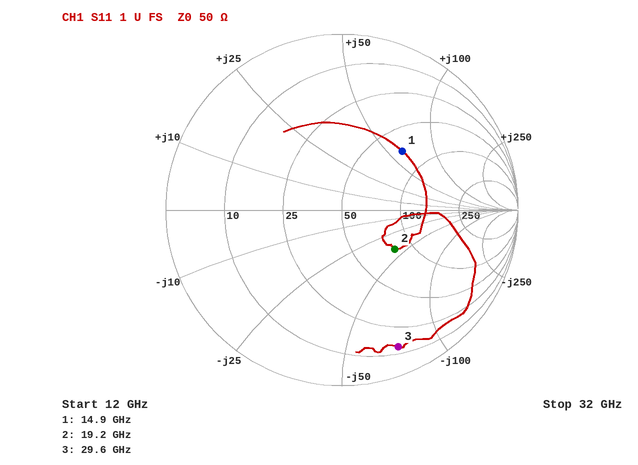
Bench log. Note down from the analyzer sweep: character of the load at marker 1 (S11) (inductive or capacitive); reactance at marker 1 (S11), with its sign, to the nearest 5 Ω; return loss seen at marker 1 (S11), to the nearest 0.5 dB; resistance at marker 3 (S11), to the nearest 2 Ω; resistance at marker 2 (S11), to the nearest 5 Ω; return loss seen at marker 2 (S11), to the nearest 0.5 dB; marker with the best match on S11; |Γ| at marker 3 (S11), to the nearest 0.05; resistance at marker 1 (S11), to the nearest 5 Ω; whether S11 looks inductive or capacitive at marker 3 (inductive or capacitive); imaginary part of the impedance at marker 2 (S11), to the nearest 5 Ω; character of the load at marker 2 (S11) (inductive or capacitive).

inductive
+60 Ω
6.5 dB
14 Ω
80 Ω
8.5 dB
marker 2
0.85
70 Ω
capacitive
-40 Ω
capacitive
